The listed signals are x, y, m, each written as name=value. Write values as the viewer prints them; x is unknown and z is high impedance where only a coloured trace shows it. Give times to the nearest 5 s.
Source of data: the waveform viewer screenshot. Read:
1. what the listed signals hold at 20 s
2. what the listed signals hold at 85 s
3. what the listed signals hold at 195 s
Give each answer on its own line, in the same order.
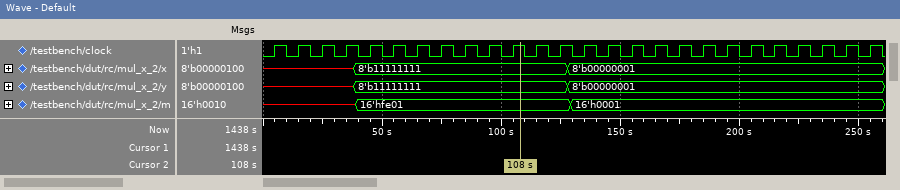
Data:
x=x, y=x, m=x
x=8'b11111111, y=8'b11111111, m=16'hfe01
x=8'b00000001, y=8'b00000001, m=16'h0001
